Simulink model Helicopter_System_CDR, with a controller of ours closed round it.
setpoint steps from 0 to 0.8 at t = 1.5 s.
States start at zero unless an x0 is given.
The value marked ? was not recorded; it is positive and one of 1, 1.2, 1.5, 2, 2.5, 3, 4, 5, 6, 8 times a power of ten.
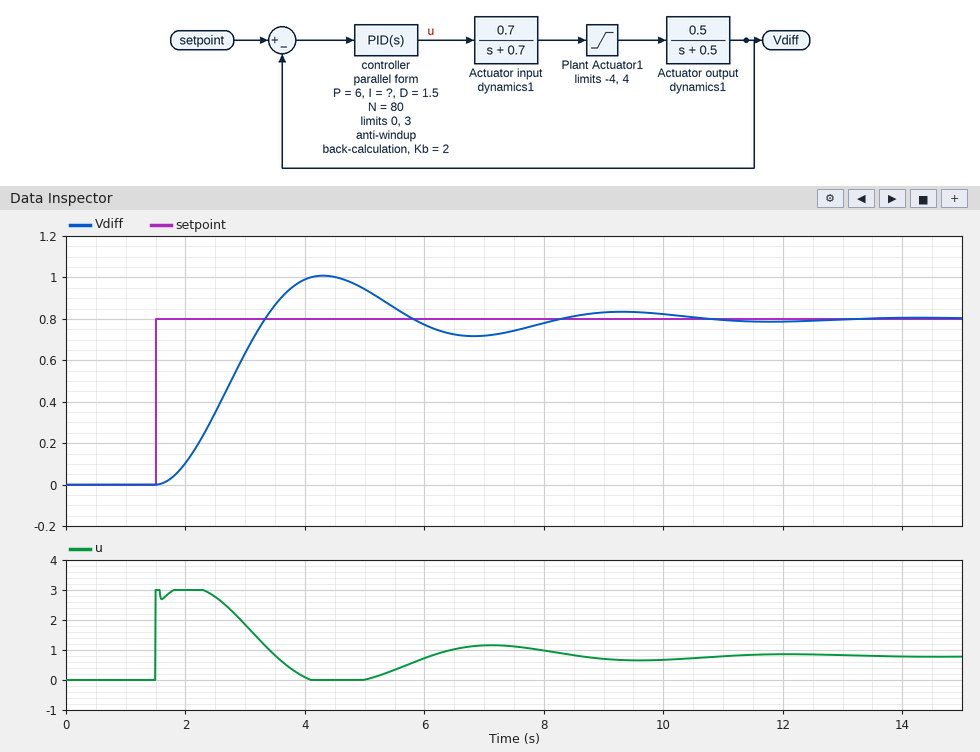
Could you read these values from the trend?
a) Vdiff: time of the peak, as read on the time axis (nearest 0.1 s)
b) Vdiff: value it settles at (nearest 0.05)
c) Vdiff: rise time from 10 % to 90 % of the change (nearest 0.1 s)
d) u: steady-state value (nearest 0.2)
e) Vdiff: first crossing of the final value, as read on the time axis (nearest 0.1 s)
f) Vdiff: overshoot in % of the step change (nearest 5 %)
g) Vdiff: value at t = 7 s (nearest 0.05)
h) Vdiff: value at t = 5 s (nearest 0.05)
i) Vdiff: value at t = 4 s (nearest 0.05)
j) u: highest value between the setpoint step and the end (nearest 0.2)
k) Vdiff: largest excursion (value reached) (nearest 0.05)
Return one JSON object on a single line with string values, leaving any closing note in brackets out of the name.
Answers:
{"Vdiff: time of the peak, as read on the time axis": "4.3 s", "Vdiff: value it settles at": "0.80", "Vdiff: rise time from 10 % to 90 % of the change": "1.2 s", "u: steady-state value": "0.8", "Vdiff: first crossing of the final value, as read on the time axis": "3.3 s", "Vdiff: overshoot in % of the step change": "25 %", "Vdiff: value at t = 7 s": "0.70", "Vdiff: value at t = 5 s": "0.95", "Vdiff: value at t = 4 s": "1.00", "u: highest value between the setpoint step and the end": "3.0", "Vdiff: largest excursion (value reached)": "1.00"}
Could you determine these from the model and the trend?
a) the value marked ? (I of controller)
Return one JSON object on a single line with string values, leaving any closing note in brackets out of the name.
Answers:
{"the value marked ?": "5"}
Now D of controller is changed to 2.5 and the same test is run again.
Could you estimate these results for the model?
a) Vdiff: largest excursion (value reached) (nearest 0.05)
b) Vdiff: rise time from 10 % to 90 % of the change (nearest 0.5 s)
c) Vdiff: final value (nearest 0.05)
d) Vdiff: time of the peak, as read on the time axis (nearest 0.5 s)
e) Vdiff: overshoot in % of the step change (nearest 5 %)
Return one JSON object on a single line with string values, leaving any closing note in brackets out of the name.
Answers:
{"Vdiff: largest excursion (value reached)": "0.95", "Vdiff: rise time from 10 % to 90 % of the change": "1.5 s", "Vdiff: final value": "0.80", "Vdiff: time of the peak, as read on the time axis": "5.0 s", "Vdiff: overshoot in % of the step change": "20 %"}
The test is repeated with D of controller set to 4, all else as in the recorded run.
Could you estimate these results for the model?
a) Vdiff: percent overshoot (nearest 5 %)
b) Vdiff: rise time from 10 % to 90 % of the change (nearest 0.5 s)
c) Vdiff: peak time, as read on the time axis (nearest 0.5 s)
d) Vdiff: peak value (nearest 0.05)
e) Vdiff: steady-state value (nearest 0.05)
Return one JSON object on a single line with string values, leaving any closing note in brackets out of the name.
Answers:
{"Vdiff: percent overshoot": "20 %", "Vdiff: rise time from 10 % to 90 % of the change": "2.0 s", "Vdiff: peak time, as read on the time axis": "6.0 s", "Vdiff: peak value": "0.95", "Vdiff: steady-state value": "0.80"}
